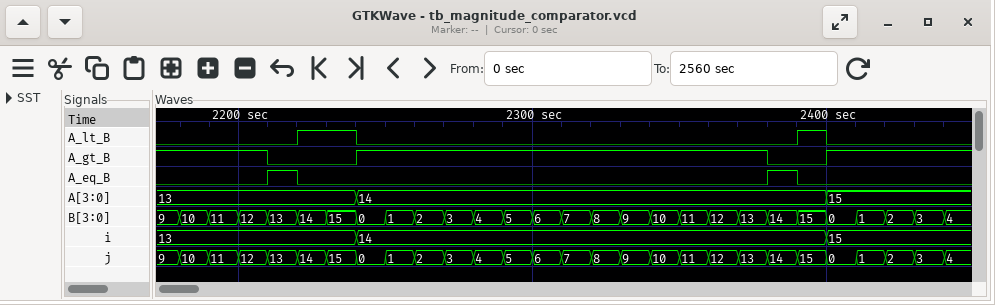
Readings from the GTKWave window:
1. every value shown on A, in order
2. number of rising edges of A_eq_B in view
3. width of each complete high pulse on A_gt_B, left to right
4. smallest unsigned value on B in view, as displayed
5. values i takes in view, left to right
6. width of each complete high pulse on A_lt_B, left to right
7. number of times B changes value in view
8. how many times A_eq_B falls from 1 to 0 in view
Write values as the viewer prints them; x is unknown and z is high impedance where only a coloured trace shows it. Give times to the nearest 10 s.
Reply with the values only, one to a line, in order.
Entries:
13, 14, 15
2
140 s
0
13, 14, 15
20 s, 10 s
27
2
